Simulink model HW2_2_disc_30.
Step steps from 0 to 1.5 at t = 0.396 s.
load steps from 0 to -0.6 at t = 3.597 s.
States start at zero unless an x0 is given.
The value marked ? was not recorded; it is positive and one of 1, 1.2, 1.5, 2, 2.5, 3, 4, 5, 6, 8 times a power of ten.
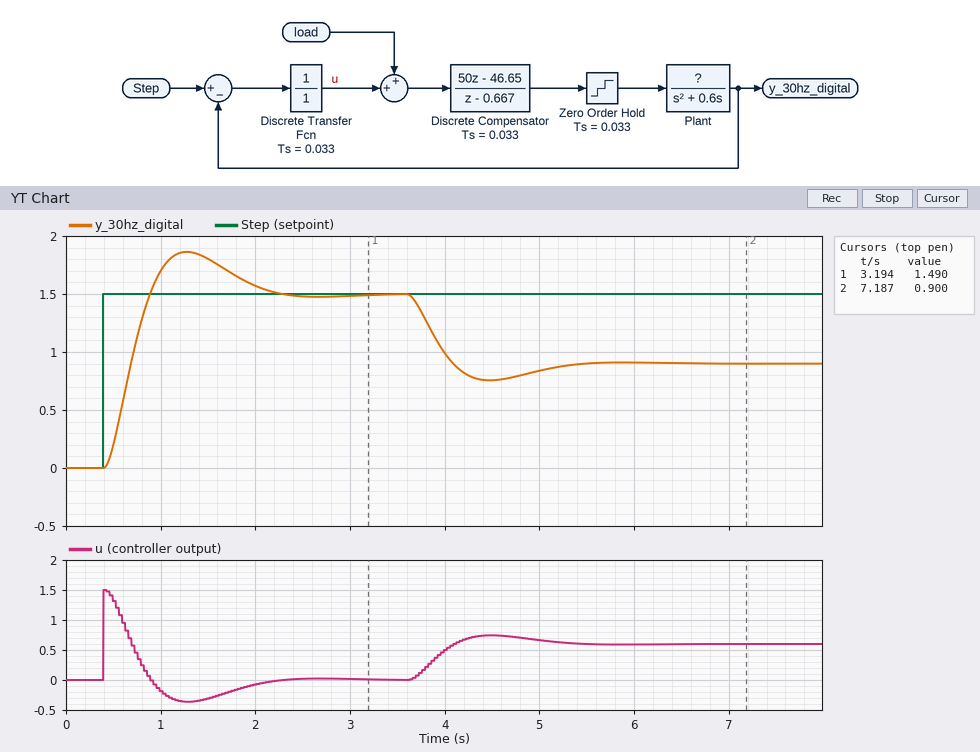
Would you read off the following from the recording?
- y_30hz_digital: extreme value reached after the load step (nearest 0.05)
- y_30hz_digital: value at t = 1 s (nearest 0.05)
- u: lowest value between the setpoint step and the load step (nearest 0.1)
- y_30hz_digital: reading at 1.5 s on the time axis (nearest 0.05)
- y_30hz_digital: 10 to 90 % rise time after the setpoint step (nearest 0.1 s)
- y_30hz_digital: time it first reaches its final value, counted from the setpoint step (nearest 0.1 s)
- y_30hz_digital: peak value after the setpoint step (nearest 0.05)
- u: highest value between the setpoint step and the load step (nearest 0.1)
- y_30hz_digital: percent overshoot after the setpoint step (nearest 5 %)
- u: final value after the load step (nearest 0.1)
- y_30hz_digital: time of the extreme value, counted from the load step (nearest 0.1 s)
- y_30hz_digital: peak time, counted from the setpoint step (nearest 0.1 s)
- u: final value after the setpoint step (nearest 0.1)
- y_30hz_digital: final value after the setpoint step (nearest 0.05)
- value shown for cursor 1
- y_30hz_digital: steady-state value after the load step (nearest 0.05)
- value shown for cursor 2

0.75
1.70
-0.4
1.80
0.3 s
0.5 s
1.85
1.5
25 %
0.6
0.9 s
0.9 s
0.0
1.50
1.490
0.90
0.900
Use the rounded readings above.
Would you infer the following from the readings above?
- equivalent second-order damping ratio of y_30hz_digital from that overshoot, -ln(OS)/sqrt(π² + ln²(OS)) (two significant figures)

0.40
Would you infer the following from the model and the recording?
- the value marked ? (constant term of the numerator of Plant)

0.6
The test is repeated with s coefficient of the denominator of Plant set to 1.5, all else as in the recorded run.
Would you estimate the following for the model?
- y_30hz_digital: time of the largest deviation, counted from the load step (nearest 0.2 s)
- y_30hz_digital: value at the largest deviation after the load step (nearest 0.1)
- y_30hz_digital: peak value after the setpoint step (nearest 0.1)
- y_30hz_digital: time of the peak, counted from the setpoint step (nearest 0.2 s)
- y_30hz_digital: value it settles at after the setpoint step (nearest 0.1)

1.0 s
0.9
1.6
1.0 s
1.5
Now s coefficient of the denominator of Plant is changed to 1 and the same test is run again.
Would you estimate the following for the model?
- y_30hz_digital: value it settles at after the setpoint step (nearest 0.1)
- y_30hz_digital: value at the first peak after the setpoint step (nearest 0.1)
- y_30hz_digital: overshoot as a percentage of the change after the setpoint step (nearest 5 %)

1.5
1.7
15 %
